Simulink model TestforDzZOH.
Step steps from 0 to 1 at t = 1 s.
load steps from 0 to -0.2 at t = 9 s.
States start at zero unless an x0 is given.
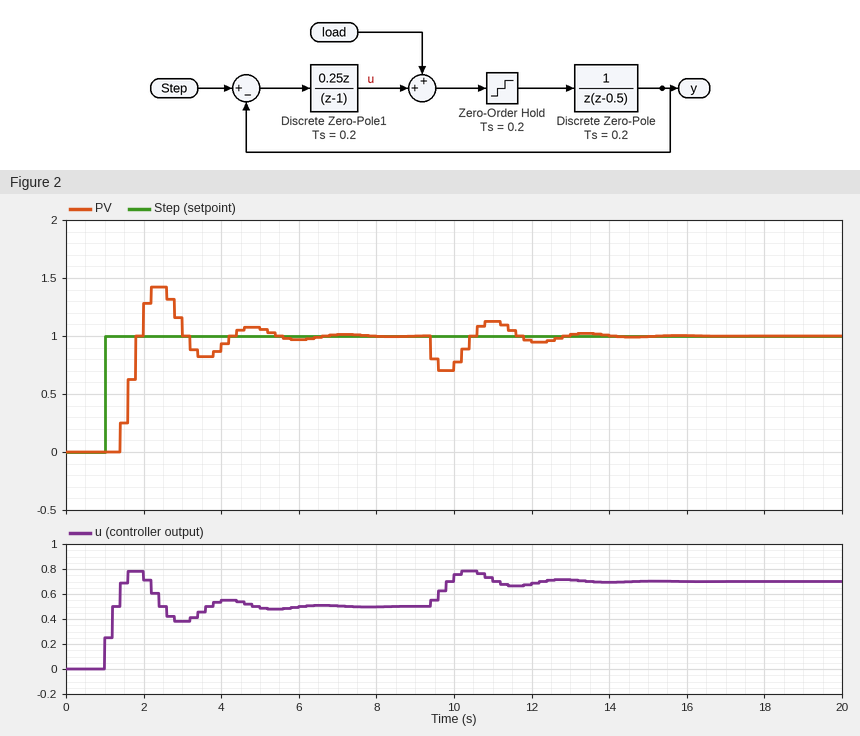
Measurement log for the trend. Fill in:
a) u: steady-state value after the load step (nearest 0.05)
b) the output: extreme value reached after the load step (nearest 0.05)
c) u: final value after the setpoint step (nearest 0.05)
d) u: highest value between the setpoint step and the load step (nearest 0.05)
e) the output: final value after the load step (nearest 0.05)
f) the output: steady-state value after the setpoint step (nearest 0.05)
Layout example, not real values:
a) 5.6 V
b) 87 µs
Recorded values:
a) 0.70
b) 0.70
c) 0.50
d) 0.80
e) 1.00
f) 1.00
